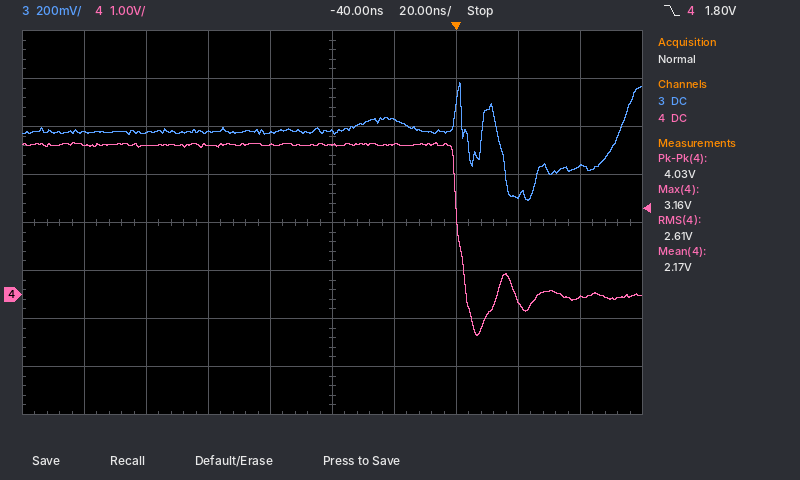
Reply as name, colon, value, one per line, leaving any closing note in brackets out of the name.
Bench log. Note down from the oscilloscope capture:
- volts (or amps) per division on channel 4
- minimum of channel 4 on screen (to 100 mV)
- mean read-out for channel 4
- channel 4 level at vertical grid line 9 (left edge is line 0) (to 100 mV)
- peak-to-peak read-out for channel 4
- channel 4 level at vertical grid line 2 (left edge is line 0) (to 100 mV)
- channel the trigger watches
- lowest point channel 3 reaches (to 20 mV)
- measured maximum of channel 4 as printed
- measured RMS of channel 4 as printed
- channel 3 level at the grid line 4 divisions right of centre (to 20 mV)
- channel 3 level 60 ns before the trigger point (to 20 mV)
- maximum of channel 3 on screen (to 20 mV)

volts (or amps) per division on channel 4: 1 V
minimum of channel 4 on screen: -900 mV
mean read-out for channel 4: 2.17 V
channel 4 level at vertical grid line 9 (left edge is line 0): -100 mV
peak-to-peak read-out for channel 4: 4.03 V
channel 4 level at vertical grid line 2 (left edge is line 0): 3.1 V
channel the trigger watches: channel 4
lowest point channel 3 reaches: 400 mV
measured maximum of channel 4 as printed: 3.16 V
measured RMS of channel 4 as printed: 2.61 V
channel 3 level at the grid line 4 divisions right of centre: 540 mV
channel 3 level 60 ns before the trigger point: 680 mV
maximum of channel 3 on screen: 880 mV
